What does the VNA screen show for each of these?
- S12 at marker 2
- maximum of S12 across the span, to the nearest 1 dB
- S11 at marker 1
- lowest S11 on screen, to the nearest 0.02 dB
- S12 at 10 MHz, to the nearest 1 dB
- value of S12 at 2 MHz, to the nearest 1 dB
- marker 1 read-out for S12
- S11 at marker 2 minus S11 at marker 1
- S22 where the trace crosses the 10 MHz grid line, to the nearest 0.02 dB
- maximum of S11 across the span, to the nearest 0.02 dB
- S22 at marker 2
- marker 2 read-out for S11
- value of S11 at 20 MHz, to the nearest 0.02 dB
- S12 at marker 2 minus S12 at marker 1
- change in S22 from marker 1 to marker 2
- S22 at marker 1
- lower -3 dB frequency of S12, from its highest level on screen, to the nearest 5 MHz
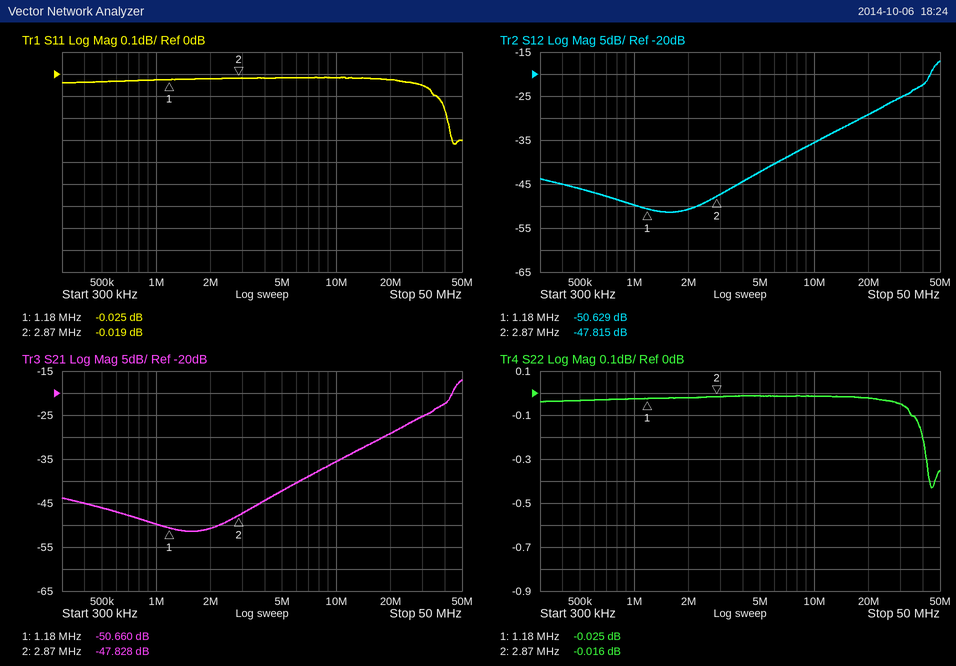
-47.815 dB
-17 dB
-0.025 dB
-0.32 dB
-36 dB
-51 dB
-50.629 dB
0.006 dB
-0.02 dB
-0.02 dB
-0.016 dB
-0.019 dB
-0.02 dB
2.814 dB
0.009 dB
-0.025 dB
45 MHz
